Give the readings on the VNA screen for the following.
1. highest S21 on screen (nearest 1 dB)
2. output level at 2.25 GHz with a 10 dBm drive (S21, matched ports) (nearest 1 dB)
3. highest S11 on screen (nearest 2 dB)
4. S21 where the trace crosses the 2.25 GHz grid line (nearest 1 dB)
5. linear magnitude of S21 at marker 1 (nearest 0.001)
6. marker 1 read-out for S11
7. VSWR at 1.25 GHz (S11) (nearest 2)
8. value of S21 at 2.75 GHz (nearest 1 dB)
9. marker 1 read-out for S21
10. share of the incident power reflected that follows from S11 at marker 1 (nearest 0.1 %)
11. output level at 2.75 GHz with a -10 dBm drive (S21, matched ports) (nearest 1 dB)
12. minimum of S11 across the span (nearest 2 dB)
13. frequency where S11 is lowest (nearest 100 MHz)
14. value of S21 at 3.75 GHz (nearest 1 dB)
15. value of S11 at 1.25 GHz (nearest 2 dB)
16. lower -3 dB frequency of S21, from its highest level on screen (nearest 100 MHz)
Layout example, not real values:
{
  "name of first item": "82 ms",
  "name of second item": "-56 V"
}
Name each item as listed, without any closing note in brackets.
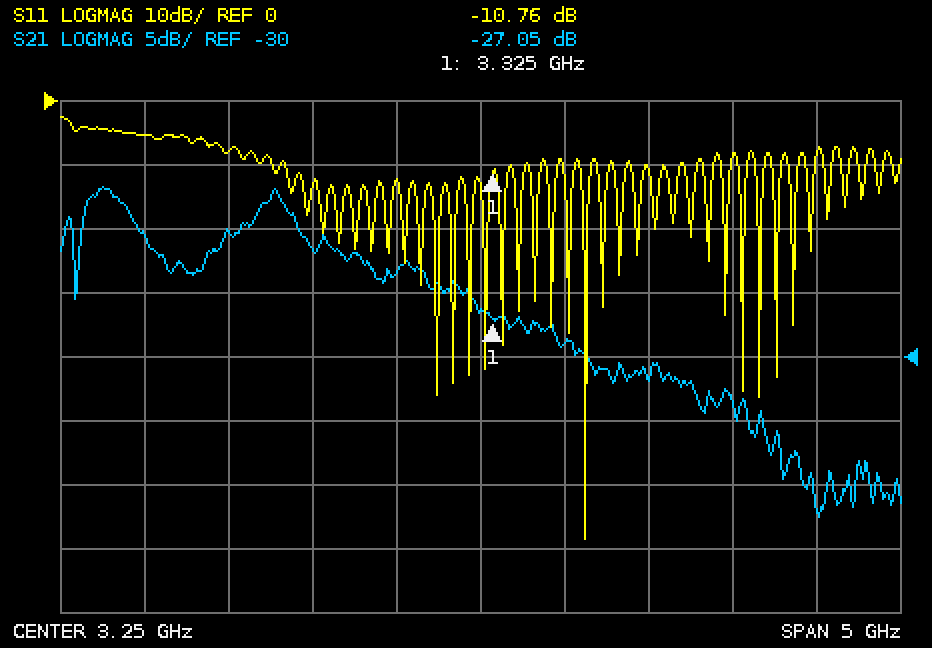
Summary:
{
  "highest S21 on screen": "-17 dB",
  "output level at 2.25 GHz with a 10 dBm drive (S21, matched ports)": "-12 dBm",
  "highest S11 on screen": "-2 dB",
  "S21 where the trace crosses the 2.25 GHz grid line": "-22 dB",
  "linear magnitude of S21 at marker 1": "0.044",
  "marker 1 read-out for S11": "-10.76 dB",
  "VSWR at 1.25 GHz (S11)": "4",
  "value of S21 at 2.75 GHz": "-23 dB",
  "marker 1 read-out for S21": "-27.05 dB",
  "share of the incident power reflected that follows from S11 at marker 1": "8.4 %",
  "output level at 2.75 GHz with a -10 dBm drive (S21, matched ports)": "-33 dBm",
  "minimum of S11 across the span": "-68 dB",
  "frequency where S11 is lowest": "3.9 GHz",
  "value of S21 at 3.75 GHz": "-29 dB",
  "value of S11 at 1.25 GHz": "-6 dB",
  "lower -3 dB frequency of S21, from its highest level on screen": "900 MHz"
}
